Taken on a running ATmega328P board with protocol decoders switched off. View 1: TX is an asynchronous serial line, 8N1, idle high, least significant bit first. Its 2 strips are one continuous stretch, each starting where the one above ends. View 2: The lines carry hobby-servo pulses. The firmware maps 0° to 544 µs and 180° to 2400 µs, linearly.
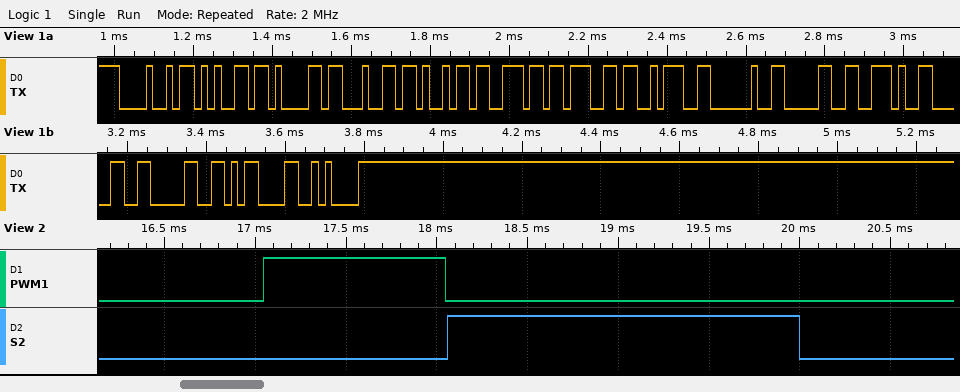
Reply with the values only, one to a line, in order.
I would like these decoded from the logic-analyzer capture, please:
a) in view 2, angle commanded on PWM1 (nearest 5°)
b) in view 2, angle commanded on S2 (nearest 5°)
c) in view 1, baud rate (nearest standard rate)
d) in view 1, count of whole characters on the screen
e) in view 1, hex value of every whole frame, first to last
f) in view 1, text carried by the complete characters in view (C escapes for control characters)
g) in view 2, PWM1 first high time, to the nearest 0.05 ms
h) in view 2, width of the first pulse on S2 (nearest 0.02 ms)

45°
135°
57600 baud
15
48 65 61 64 69 6E 67 3A 20 30 2E 30 30 0D 0A
"Heading: 0.00\r\n"
1.00 ms
1.94 ms
